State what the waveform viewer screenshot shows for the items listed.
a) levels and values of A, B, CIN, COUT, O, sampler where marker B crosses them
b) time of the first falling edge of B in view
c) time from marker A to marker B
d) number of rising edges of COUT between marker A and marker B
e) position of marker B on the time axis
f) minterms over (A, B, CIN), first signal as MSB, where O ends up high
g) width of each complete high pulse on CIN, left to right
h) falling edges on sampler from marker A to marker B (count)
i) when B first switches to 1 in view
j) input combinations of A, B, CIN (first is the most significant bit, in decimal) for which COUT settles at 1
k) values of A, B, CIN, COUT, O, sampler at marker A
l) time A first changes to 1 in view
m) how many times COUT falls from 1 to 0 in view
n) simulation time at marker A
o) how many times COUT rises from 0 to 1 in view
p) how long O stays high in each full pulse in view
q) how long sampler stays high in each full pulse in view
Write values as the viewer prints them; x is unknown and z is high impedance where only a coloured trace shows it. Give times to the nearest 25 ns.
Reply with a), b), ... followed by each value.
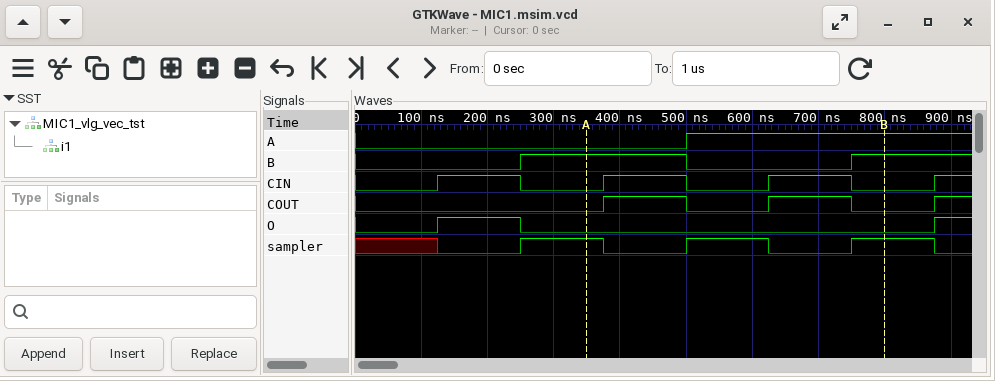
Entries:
a) A=1, B=1, CIN=0, COUT=0, O=0, sampler=1
b) 500 ns
c) 450 ns
d) 2
e) 800 ns
f) 1, 7
g) 125 ns, 125 ns, 125 ns
h) 2
i) 250 ns
j) 3, 5, 7
k) A=0, B=1, CIN=0, COUT=0, O=0, sampler=1
l) 500 ns
m) 2
n) 350 ns
o) 3
p) 125 ns
q) 125 ns, 125 ns, 125 ns
